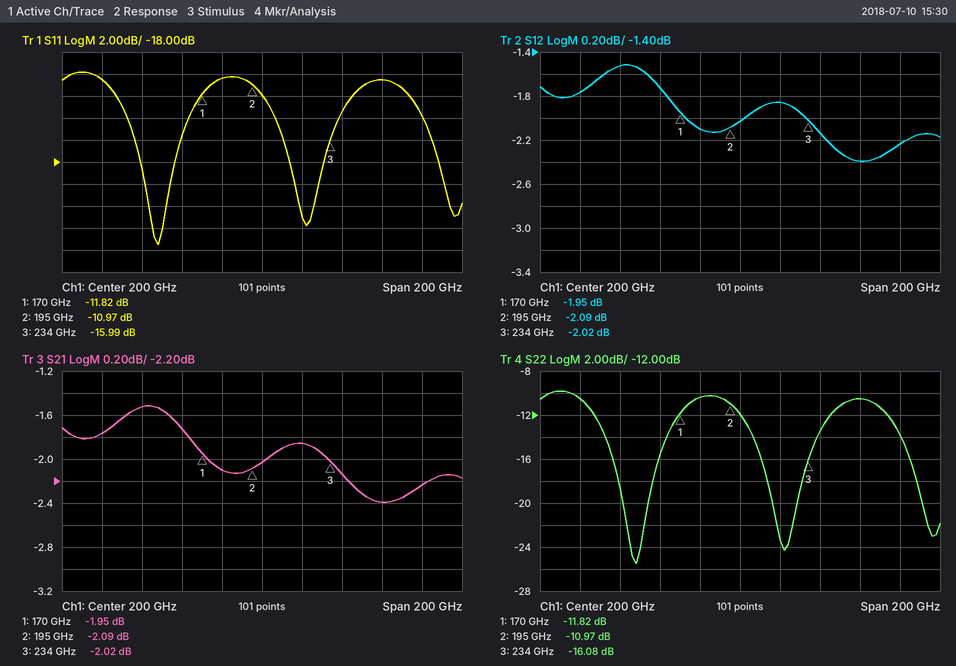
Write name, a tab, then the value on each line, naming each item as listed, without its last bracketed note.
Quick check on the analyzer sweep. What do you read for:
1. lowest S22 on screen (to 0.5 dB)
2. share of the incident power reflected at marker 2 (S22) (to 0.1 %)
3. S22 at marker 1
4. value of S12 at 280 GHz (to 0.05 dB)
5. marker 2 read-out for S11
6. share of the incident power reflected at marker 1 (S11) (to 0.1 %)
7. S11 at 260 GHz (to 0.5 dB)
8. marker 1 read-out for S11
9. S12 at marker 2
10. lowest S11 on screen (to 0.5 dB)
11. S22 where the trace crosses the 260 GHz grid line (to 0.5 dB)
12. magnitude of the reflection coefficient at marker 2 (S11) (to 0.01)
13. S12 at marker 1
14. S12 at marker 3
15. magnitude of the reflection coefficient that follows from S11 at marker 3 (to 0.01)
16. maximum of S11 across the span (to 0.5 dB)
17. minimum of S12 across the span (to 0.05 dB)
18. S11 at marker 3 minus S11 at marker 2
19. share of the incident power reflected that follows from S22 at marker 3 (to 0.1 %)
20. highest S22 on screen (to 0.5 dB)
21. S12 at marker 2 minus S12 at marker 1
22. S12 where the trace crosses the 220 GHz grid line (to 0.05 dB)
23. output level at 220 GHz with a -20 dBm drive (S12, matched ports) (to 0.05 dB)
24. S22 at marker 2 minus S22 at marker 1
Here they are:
lowest S22 on screen	-25.5 dB
share of the incident power reflected at marker 2 (S22)	8.0 %
S22 at marker 1	-11.82 dB
value of S12 at 280 GHz	-2.25 dB
marker 2 read-out for S11	-10.97 dB
share of the incident power reflected at marker 1 (S11)	6.6 %
S11 at 260 GHz	-10.5 dB
marker 1 read-out for S11	-11.82 dB
S12 at marker 2	-2.09 dB
lowest S11 on screen	-25.5 dB
S22 where the trace crosses the 260 GHz grid line	-10.5 dB
magnitude of the reflection coefficient at marker 2 (S11)	0.28
S12 at marker 1	-1.95 dB
S12 at marker 3	-2.02 dB
magnitude of the reflection coefficient that follows from S11 at marker 3	0.16
maximum of S11 across the span	-10.0 dB
minimum of S12 across the span	-2.40 dB
S11 at marker 3 minus S11 at marker 2	-5.02 dB
share of the incident power reflected that follows from S22 at marker 3	2.5 %
highest S22 on screen	-10.0 dB
S12 at marker 2 minus S12 at marker 1	-0.14 dB
S12 where the trace crosses the 220 GHz grid line	-1.85 dB
output level at 220 GHz with a -20 dBm drive (S12, matched ports)	-21.85 dBm
S22 at marker 2 minus S22 at marker 1	0.85 dB
